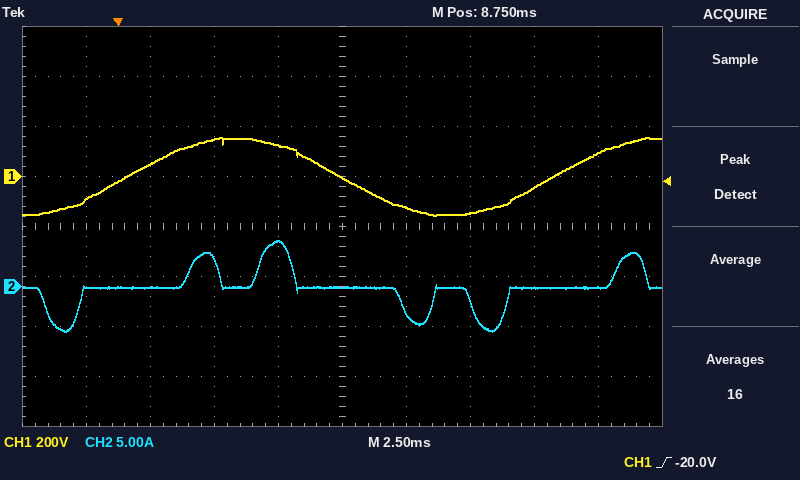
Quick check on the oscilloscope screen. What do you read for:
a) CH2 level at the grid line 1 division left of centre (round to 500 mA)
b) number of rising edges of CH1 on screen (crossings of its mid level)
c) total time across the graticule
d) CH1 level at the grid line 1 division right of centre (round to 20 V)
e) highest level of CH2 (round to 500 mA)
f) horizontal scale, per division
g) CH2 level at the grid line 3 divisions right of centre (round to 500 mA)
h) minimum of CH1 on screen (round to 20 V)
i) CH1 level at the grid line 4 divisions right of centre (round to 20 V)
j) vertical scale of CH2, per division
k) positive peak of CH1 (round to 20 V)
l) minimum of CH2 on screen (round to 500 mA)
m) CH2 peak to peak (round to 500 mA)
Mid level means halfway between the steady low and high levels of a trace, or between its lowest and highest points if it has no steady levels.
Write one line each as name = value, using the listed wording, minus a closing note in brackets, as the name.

CH2 level at the grid line 1 division left of centre = 4.5 A
number of rising edges of CH1 on screen = 2
total time across the graticule = 25 ms
CH1 level at the grid line 1 division right of centre = -120 V
highest level of CH2 = 4.5 A
horizontal scale, per division = 2.5 ms
CH2 level at the grid line 3 divisions right of centre = 0.0 A
minimum of CH1 on screen = -160 V
CH1 level at the grid line 4 divisions right of centre = 100 V
vertical scale of CH2, per division = 5 A
positive peak of CH1 = 160 V
minimum of CH2 on screen = -4.5 A
CH2 peak to peak = 9.0 A
